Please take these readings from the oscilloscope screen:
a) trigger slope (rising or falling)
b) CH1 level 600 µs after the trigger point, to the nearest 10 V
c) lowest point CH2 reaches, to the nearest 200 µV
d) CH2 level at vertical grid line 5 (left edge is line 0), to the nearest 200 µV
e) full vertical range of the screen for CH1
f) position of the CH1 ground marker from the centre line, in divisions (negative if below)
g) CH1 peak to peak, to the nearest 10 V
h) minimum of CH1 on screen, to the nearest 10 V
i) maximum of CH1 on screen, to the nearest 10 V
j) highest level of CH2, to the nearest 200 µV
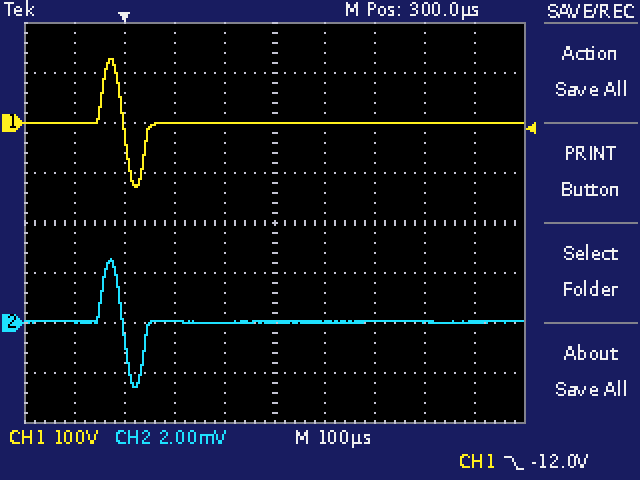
falling
0 V
-2.6 mV
0.0 mV
800 V
+2.0 div
260 V
-130 V
130 V
2.6 mV
